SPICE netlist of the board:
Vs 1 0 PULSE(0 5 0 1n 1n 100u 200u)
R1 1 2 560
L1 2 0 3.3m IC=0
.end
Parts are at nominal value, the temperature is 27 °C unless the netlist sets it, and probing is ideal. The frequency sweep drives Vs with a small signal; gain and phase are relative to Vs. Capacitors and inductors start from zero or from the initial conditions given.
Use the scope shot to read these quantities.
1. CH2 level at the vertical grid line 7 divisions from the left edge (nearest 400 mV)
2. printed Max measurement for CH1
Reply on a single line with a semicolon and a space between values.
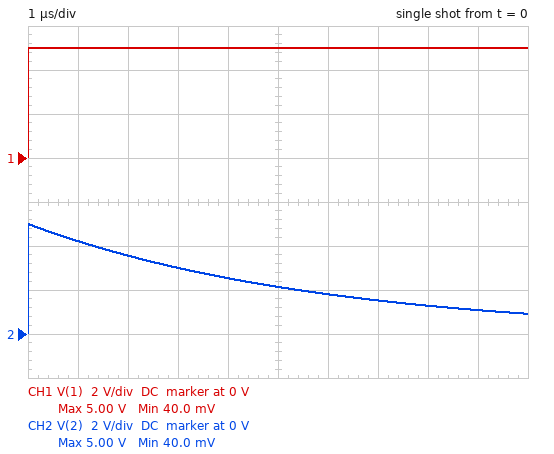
1.6 V; 5.00 V
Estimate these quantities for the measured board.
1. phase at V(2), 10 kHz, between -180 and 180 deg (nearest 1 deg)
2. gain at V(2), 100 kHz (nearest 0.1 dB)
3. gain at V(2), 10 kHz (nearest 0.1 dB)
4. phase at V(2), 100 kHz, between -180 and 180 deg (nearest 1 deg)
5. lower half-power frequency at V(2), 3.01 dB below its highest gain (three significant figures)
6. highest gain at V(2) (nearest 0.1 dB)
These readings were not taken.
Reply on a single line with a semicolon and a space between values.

70 deg; -0.3 dB; -9.2 dB; 15 deg; 27.0 kHz; 0 dB
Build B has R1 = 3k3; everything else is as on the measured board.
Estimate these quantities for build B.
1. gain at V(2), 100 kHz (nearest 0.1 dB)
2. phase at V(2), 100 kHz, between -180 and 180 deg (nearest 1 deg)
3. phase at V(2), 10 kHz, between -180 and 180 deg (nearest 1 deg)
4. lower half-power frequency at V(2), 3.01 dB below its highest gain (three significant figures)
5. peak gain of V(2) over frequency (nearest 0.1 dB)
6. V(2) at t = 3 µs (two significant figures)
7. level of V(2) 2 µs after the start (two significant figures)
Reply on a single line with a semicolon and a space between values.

-5.5 dB; 58 deg; 86 deg; 159 kHz; 0 dB; 250 mV; 680 mV
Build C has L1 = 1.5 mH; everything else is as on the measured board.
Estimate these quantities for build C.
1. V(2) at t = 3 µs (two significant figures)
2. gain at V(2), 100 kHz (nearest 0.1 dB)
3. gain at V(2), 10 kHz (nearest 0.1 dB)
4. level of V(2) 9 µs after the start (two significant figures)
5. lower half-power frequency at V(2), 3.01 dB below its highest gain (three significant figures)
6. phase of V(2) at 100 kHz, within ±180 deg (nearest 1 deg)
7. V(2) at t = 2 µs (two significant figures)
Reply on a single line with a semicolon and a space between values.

1.6 V; -1.3 dB; -15.6 dB; 170 mV; 59.4 kHz; 31 deg; 2.4 V
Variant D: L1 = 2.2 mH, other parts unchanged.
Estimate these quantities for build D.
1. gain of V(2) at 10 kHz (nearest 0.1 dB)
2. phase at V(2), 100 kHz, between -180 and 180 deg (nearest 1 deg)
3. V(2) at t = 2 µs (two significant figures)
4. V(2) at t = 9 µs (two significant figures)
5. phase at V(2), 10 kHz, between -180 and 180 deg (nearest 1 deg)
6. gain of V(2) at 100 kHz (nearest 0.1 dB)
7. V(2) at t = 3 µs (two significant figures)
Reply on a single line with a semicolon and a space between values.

-12.4 dB; 22 deg; 3.0 V; 510 mV; 76 deg; -0.7 dB; 2.3 V
